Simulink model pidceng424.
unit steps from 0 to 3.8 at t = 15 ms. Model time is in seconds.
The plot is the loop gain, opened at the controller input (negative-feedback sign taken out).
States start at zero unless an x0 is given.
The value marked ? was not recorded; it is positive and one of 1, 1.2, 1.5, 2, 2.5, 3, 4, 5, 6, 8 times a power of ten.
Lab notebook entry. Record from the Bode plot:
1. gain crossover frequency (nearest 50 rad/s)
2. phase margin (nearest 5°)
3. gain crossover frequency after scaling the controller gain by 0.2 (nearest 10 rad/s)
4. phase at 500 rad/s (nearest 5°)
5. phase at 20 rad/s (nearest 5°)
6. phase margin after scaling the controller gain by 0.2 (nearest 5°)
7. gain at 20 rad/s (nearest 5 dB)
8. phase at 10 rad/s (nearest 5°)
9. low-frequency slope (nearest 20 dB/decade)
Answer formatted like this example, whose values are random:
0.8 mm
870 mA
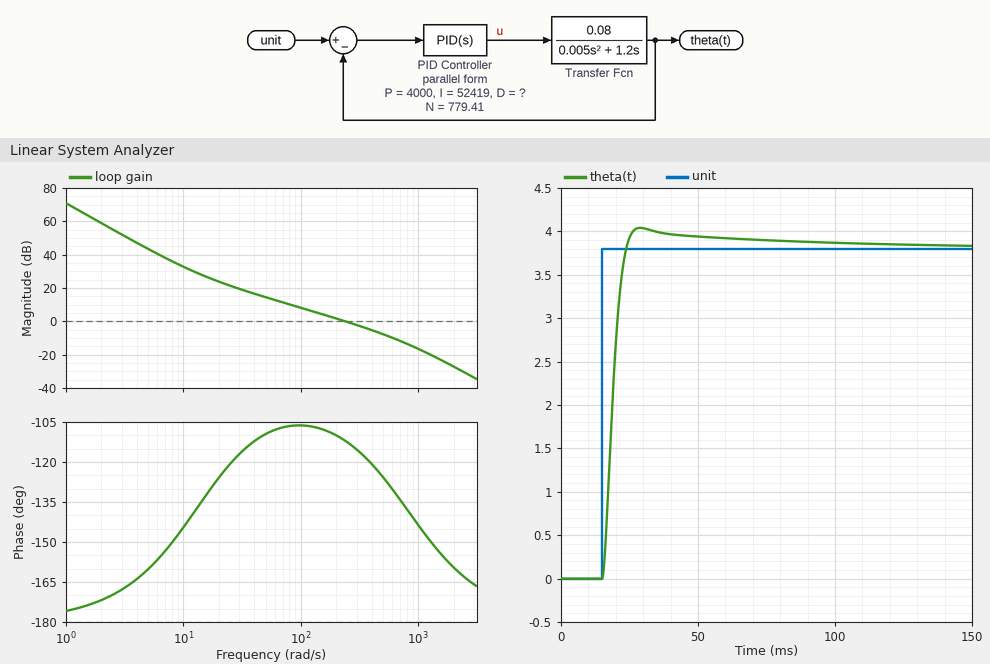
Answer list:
250 rad/s
70°
50 rad/s
-125°
-125°
70°
25 dB
-145°
-40 dB/decade
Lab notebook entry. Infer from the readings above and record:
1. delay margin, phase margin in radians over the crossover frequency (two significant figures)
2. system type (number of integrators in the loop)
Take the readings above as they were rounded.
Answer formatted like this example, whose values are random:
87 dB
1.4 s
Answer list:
0.0049 s
2
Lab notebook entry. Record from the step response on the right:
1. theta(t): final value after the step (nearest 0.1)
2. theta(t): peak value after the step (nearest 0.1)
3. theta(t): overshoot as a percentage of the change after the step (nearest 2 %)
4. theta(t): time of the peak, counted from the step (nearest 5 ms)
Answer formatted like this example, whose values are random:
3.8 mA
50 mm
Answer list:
3.8
4.0
6 %
15 ms
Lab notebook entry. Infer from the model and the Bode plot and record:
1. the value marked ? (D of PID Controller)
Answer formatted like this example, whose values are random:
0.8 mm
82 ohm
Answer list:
10
